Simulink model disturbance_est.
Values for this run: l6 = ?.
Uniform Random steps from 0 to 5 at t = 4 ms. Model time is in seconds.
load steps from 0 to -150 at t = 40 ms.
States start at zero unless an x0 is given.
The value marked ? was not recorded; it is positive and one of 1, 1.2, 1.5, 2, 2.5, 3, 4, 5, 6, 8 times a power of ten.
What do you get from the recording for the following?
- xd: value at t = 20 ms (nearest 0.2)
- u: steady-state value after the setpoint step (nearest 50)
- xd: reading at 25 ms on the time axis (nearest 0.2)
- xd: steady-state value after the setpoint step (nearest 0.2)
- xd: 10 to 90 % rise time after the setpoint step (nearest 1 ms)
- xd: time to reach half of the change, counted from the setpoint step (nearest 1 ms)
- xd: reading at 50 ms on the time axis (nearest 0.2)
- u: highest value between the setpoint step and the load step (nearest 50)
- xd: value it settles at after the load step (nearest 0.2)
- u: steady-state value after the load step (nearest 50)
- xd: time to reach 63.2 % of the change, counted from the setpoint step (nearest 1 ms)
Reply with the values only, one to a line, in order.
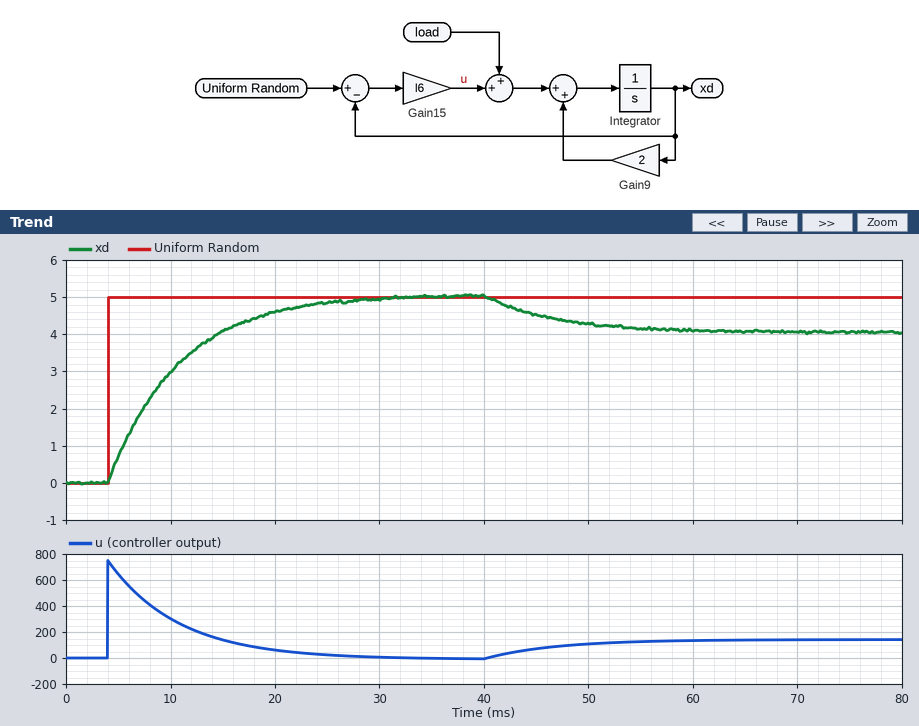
4.6
0
4.8
5.0
15 ms
5 ms
4.2
750
4.0
150
7 ms
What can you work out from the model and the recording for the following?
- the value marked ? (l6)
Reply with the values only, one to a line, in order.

150
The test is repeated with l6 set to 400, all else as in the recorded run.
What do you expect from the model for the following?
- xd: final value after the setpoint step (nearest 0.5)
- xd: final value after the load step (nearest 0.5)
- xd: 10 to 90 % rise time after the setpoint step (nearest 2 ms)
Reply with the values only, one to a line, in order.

5.0
4.5
6 ms
